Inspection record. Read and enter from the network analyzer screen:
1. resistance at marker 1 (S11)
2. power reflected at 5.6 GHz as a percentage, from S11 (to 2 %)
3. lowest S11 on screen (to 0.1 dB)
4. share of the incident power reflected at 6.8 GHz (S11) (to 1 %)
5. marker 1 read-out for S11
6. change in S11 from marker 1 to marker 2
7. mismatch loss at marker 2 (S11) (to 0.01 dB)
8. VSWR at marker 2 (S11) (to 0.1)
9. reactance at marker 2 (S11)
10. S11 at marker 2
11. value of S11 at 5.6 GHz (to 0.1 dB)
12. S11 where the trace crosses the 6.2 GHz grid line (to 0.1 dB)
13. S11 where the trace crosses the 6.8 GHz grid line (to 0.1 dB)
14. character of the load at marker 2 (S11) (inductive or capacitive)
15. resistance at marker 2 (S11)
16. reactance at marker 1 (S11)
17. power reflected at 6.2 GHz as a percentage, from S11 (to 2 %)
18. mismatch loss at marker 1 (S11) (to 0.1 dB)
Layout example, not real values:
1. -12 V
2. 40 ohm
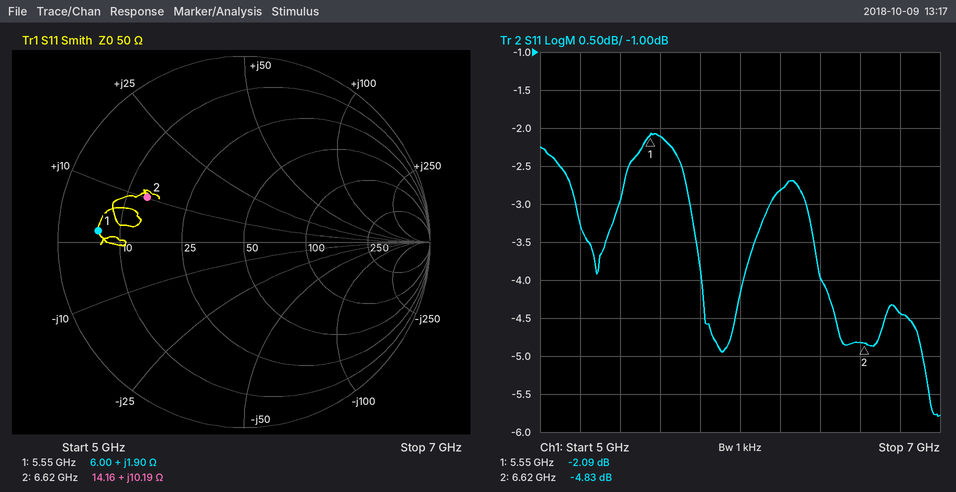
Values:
1. 6.00 Ω
2. 62 %
3. -5.8 dB
4. 36 %
5. -2.09 dB
6. -2.74 dB
7. 1.73 dB
8. 3.7
9. +10.19 Ω
10. -4.83 dB
11. -2.1 dB
12. -2.8 dB
13. -4.4 dB
14. inductive
15. 14.16 Ω
16. +1.90 Ω
17. 52 %
18. 4.2 dB
